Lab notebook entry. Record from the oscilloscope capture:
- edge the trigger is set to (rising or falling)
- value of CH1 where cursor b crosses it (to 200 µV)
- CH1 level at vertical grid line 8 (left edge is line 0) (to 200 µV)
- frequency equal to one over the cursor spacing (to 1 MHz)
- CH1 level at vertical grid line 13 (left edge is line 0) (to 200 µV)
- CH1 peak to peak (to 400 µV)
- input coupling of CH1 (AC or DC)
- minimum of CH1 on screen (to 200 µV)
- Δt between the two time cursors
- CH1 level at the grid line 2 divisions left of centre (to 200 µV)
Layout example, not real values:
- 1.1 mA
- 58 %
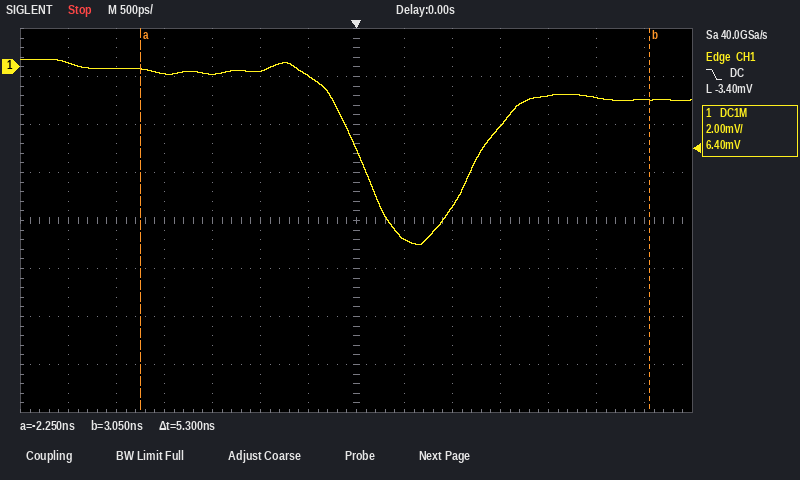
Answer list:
- falling
- -1.4 mV
- -7.2 mV
- 189 MHz
- -1.4 mV
- 7.6 mV
- DC
- -7.4 mV
- 5.3 ns
- -200 µV
